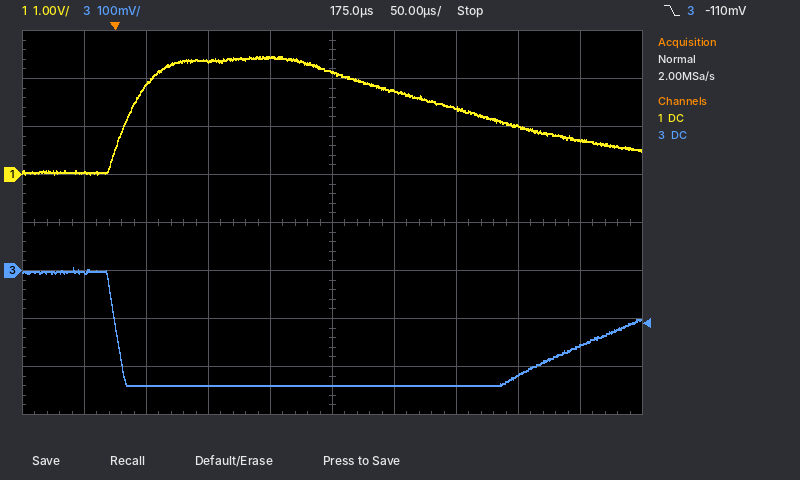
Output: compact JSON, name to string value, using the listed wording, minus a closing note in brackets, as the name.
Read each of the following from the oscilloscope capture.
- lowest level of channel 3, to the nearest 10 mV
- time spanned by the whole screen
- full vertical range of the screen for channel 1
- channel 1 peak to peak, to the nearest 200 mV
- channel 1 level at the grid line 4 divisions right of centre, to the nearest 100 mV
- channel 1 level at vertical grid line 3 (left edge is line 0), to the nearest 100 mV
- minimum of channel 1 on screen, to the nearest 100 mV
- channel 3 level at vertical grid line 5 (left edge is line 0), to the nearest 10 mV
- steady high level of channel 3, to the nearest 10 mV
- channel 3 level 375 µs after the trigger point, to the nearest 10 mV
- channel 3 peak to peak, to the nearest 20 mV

{"lowest level of channel 3, to the nearest 10 mV": "-240 mV", "time spanned by the whole screen": "500 µs", "full vertical range of the screen for channel 1": "8 V", "channel 1 peak to peak, to the nearest 200 mV": "2.4 V", "channel 1 level at the grid line 4 divisions right of centre, to the nearest 100 mV": "700 mV", "channel 1 level at vertical grid line 3 (left edge is line 0), to the nearest 100 mV": "2.4 V", "minimum of channel 1 on screen, to the nearest 100 mV": "0.0 V", "channel 3 level at vertical grid line 5 (left edge is line 0), to the nearest 10 mV": "-240 mV", "steady high level of channel 3, to the nearest 10 mV": "0 mV", "channel 3 level 375 µs after the trigger point, to the nearest 10 mV": "-160 mV", "channel 3 peak to peak, to the nearest 20 mV": "240 mV"}
